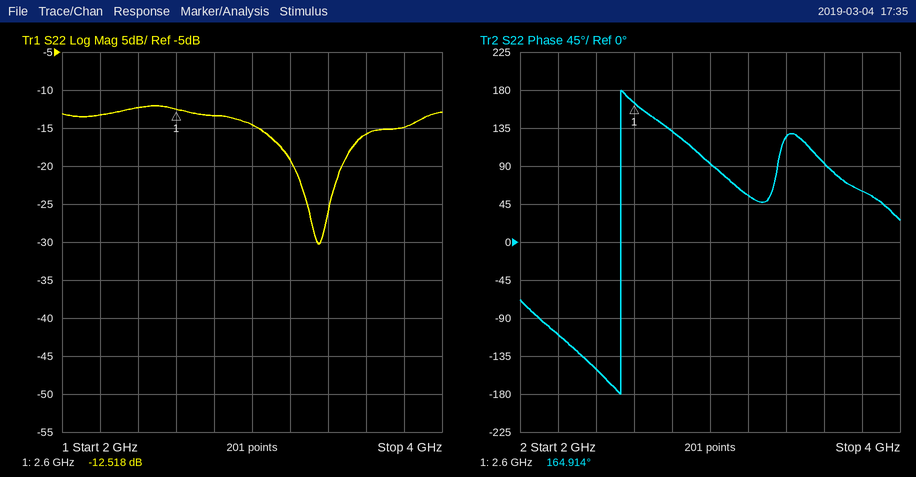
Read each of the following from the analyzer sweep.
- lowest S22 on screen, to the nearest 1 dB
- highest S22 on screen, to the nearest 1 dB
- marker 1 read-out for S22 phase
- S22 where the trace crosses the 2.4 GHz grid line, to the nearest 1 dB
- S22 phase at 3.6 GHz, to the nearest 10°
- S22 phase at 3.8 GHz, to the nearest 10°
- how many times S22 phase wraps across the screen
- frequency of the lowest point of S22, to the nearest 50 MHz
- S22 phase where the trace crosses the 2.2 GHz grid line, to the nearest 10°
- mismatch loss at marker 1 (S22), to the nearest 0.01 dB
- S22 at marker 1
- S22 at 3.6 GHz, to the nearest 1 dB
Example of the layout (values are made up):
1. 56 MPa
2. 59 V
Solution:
1. -30 dB
2. -12 dB
3. 164.914°
4. -12 dB
5. 90°
6. 60°
7. 1
8. 3.35 GHz
9. -110°
10. 0.25 dB
11. -12.518 dB
12. -16 dB
